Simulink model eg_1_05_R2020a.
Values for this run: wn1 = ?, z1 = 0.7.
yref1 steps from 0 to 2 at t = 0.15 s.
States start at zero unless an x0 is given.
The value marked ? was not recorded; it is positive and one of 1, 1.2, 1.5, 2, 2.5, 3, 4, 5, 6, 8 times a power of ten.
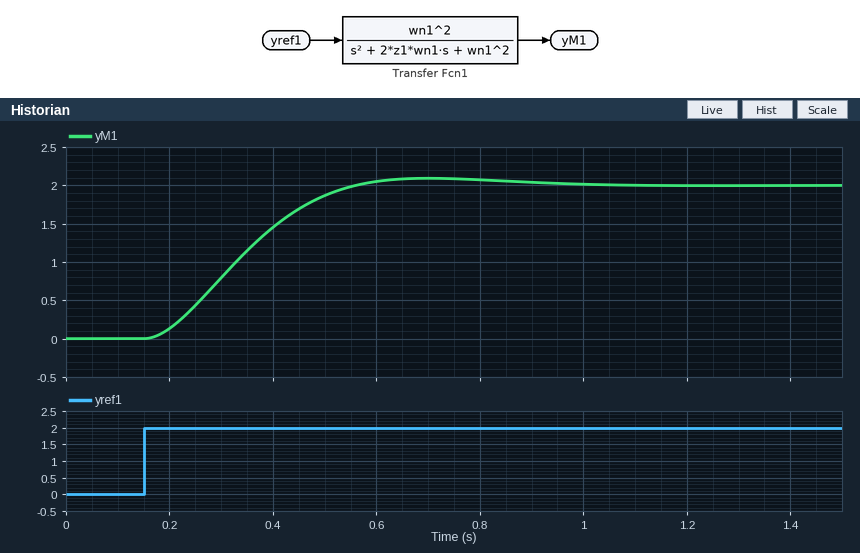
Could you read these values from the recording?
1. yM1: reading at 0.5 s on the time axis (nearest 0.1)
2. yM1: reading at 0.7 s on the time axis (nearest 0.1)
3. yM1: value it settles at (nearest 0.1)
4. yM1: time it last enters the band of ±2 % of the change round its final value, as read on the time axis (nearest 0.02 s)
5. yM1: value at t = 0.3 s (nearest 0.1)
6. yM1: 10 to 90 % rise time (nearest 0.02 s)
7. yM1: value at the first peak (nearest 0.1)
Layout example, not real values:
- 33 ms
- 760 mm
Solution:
- 1.9
- 2.1
- 2.0
- 0.90 s
- 0.8
- 0.26 s
- 2.1
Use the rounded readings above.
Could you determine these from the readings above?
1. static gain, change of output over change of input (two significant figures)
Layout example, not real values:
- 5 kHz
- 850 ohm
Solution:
- 1.0
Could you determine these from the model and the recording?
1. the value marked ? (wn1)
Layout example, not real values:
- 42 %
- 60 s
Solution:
- 8
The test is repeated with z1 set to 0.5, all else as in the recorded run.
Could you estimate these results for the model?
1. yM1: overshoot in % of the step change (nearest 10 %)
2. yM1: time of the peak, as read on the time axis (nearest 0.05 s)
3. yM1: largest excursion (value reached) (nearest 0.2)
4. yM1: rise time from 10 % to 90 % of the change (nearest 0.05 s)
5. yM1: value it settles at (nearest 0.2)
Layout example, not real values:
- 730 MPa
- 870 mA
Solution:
- 20 %
- 0.60 s
- 2.4
- 0.20 s
- 2.0
